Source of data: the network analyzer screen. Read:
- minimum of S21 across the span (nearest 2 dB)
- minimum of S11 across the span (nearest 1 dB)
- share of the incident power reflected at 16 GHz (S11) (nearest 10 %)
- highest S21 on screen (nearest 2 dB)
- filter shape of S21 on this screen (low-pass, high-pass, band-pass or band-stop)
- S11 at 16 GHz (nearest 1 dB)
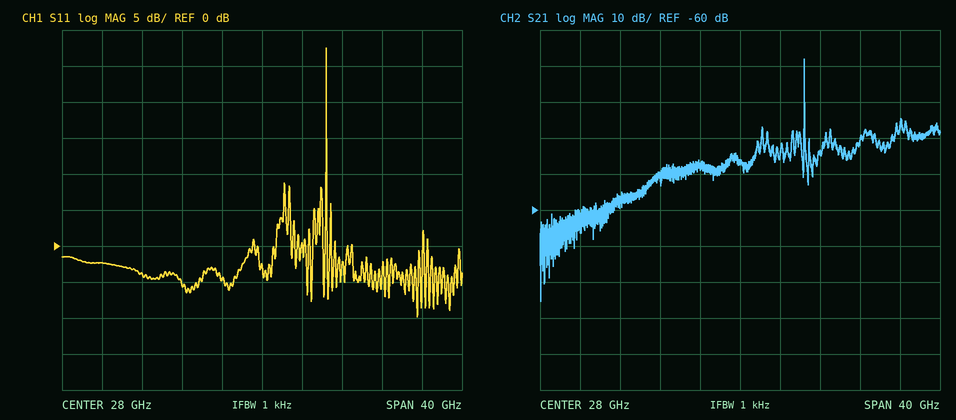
-86 dB
-10 dB
40 %
-18 dB
band-pass
-4 dB
